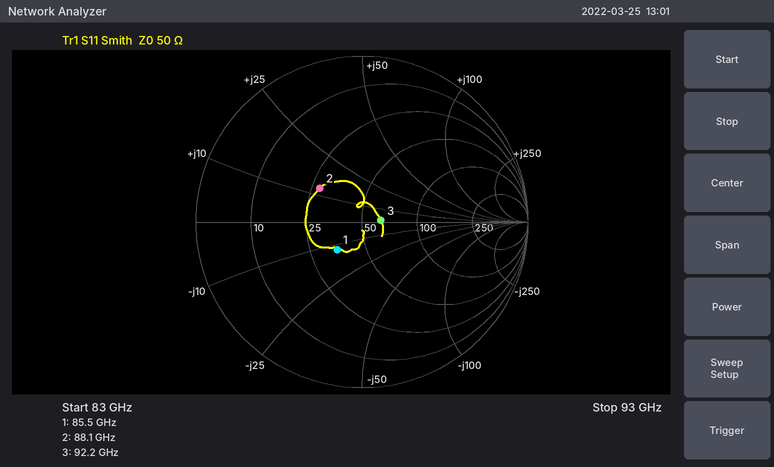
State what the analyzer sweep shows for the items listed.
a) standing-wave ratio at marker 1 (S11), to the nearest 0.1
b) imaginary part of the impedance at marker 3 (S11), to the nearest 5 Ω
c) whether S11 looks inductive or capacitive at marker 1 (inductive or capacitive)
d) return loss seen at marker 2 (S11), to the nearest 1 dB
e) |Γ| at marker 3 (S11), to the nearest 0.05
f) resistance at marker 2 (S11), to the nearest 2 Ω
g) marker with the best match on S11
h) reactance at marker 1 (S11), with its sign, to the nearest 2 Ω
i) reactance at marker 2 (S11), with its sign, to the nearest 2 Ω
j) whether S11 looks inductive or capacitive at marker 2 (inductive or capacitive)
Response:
1.6
0 Ω
capacitive
10 dB
0.10
28 Ω
marker 3
-12 Ω
+12 Ω
inductive
